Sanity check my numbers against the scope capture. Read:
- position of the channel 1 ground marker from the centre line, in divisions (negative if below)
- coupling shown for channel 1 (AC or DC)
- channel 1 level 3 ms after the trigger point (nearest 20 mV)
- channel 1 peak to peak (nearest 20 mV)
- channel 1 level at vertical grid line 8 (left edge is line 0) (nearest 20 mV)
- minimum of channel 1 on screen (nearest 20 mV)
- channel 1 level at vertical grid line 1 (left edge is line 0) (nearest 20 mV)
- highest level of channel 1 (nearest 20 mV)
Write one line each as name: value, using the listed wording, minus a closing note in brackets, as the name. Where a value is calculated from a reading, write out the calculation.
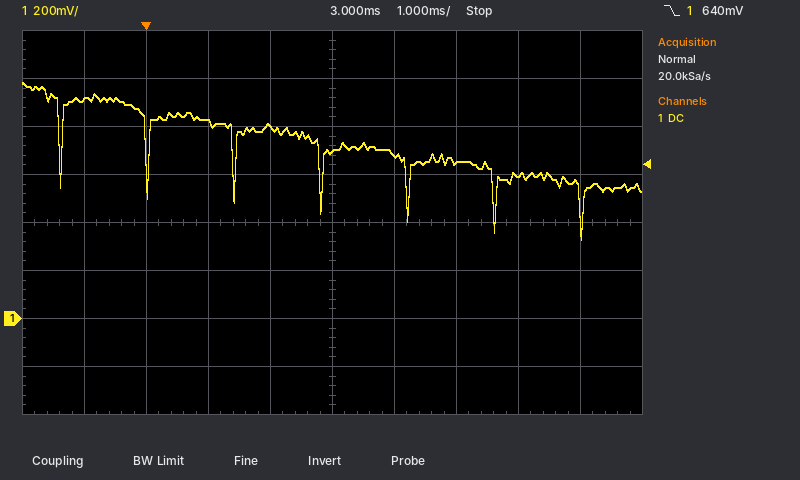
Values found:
position of the channel 1 ground marker from the centre line, in divisions: -2.0 div
coupling shown for channel 1: DC
channel 1 level 3 ms after the trigger point: 700 mV
channel 1 peak to peak: 980 mV − (320 mV) = 660 mV
channel 1 level at vertical grid line 8 (left edge is line 0): 600 mV
minimum of channel 1 on screen: 320 mV
channel 1 level at vertical grid line 1 (left edge is line 0): 920 mV
highest level of channel 1: 980 mV
